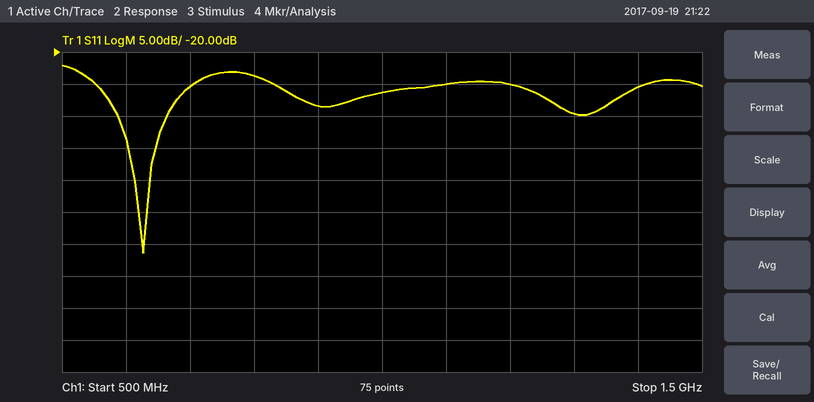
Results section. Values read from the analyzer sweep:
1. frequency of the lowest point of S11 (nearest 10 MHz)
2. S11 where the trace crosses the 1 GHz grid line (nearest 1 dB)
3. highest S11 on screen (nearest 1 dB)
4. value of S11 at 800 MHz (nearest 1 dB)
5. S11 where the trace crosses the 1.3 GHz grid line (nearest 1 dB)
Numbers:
630 MHz
-26 dB
-22 dB
-24 dB
-30 dB
